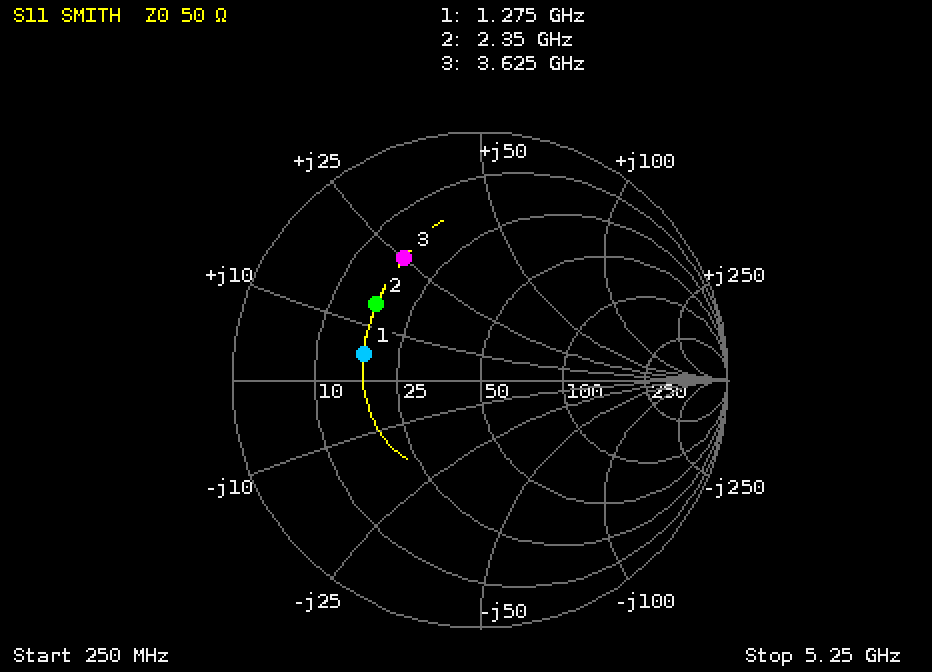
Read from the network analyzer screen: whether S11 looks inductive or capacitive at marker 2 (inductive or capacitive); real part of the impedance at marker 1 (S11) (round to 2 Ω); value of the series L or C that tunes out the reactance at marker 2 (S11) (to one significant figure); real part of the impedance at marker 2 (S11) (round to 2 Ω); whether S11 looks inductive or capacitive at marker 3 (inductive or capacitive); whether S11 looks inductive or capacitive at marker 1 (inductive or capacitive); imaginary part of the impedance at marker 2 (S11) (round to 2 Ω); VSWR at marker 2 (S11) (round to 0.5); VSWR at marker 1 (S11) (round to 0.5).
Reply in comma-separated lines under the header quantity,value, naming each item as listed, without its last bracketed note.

quantity,value
whether S11 looks inductive or capacitive at marker 2,inductive
real part of the impedance at marker 1 (S11),18 Ω
value of the series L or C that tunes out the reactance at marker 2 (S11),5 pF
real part of the impedance at marker 2 (S11),18 Ω
whether S11 looks inductive or capacitive at marker 3,inductive
whether S11 looks inductive or capacitive at marker 1,inductive
imaginary part of the impedance at marker 2 (S11),+14 Ω
VSWR at marker 2 (S11),3.0
VSWR at marker 1 (S11),3.0
